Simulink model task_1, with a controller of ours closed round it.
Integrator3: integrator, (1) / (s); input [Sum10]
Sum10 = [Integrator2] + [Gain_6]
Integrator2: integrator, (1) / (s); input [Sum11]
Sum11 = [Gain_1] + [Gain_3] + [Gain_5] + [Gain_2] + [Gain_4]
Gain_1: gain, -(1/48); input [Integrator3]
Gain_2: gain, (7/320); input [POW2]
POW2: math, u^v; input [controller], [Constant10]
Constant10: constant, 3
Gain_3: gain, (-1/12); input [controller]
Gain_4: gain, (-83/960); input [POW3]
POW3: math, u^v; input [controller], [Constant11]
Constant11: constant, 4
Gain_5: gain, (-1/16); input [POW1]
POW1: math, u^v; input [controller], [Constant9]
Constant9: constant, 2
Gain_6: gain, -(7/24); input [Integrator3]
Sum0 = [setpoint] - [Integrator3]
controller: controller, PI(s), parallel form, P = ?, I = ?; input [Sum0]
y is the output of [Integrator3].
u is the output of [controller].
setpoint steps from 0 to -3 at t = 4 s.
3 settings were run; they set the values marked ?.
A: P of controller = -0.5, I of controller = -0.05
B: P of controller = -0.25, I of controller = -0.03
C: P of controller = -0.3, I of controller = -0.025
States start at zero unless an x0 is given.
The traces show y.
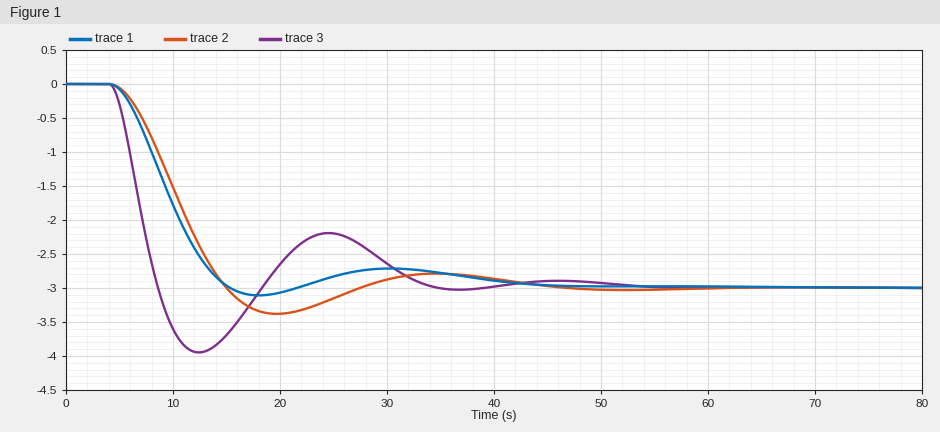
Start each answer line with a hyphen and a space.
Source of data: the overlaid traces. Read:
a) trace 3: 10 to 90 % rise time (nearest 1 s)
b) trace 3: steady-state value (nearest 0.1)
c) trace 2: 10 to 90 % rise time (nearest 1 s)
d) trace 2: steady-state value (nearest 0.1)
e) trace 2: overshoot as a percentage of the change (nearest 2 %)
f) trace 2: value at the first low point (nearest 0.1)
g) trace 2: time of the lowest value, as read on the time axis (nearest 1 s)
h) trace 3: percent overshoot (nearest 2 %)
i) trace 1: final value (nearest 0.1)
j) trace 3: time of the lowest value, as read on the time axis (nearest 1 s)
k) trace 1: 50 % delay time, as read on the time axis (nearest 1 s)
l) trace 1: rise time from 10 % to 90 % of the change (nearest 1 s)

- 3 s
- -3.0
- 7 s
- -3.0
- 12 %
- -3.4
- 20 s
- 32 %
- -3.0
- 12 s
- 9 s
- 7 s
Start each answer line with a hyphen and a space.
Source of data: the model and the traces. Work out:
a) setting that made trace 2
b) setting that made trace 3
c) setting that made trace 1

- B
- A
- C
